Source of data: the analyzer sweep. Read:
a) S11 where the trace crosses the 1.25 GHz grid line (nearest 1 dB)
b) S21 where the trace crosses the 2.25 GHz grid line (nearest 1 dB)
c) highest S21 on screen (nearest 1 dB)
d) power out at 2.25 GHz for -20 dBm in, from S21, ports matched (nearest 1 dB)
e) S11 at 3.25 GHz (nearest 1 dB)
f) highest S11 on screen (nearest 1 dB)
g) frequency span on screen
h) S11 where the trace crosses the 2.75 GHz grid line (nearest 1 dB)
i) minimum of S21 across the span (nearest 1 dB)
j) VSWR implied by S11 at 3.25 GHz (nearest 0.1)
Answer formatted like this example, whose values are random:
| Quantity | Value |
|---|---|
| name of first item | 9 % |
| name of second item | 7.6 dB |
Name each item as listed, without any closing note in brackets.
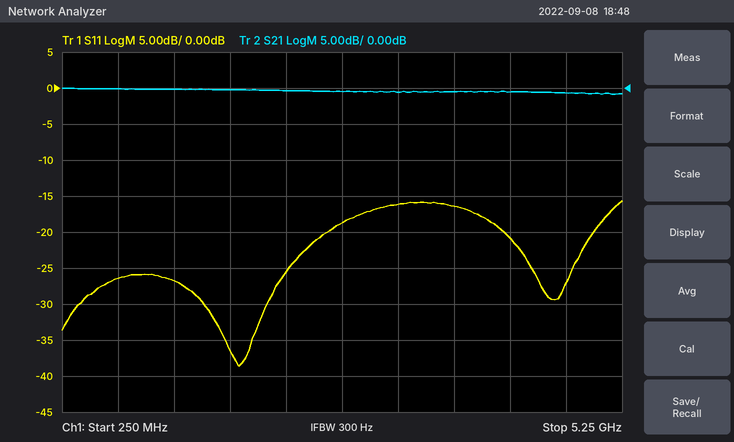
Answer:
| Quantity | Value |
|---|---|
| S11 where the trace crosses the 1.25 GHz grid line | -27 dB |
| S21 where the trace crosses the 2.25 GHz grid line | 0 dB |
| highest S21 on screen | 0 dB |
| power out at 2.25 GHz for -20 dBm in, from S21, ports matched | -20 dBm |
| S11 at 3.25 GHz | -16 dB |
| highest S11 on screen | -16 dB |
| frequency span on screen | 5 GHz |
| S11 where the trace crosses the 2.75 GHz grid line | -19 dB |
| minimum of S21 across the span | -1 dB |
| VSWR implied by S11 at 3.25 GHz | 1.4 |
